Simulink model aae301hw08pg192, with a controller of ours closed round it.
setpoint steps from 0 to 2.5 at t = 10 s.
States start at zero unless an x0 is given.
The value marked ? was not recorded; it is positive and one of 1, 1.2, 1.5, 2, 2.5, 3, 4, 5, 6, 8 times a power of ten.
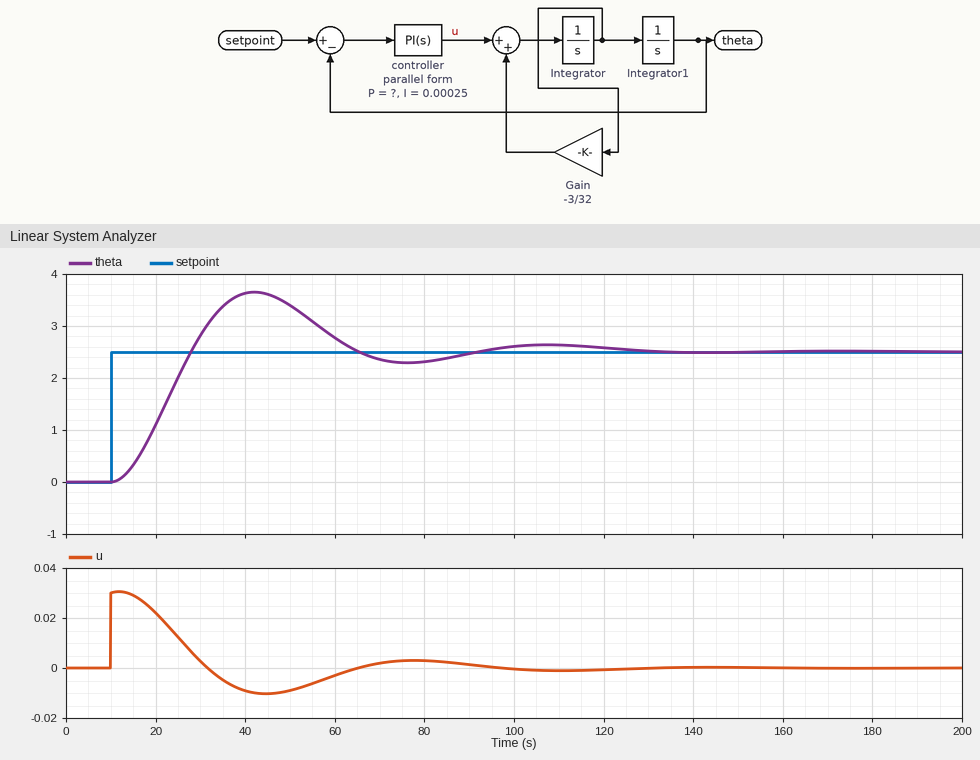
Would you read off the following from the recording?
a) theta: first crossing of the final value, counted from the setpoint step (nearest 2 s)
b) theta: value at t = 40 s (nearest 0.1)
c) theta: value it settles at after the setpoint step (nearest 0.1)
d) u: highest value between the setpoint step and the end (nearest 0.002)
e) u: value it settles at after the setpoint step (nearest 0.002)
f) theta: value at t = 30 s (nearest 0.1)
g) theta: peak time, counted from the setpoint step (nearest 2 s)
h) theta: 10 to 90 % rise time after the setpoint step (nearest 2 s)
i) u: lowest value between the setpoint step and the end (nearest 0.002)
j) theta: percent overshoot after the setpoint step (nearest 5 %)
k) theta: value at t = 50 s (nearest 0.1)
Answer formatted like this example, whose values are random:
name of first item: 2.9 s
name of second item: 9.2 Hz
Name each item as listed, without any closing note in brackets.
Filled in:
theta: first crossing of the final value, counted from the setpoint step: 18 s
theta: value at t = 40 s: 3.6
theta: value it settles at after the setpoint step: 2.5
u: highest value between the setpoint step and the end: 0.030
u: value it settles at after the setpoint step: 0.000
theta: value at t = 30 s: 2.8
theta: peak time, counted from the setpoint step: 32 s
theta: 10 to 90 % rise time after the setpoint step: 12 s
u: lowest value between the setpoint step and the end: -0.010
theta: percent overshoot after the setpoint step: 45 %
theta: value at t = 50 s: 3.4
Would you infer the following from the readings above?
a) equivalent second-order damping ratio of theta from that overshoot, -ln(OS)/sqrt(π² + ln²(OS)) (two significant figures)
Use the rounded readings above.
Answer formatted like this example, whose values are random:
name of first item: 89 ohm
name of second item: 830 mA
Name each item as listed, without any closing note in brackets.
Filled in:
equivalent second-order damping ratio of theta from that overshoot, -ln(OS)/sqrt(π² + ln²(OS)): 0.25
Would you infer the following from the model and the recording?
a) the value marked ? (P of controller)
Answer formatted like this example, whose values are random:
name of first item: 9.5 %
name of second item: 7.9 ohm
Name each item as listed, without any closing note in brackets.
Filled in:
the value marked ?: 0.012
